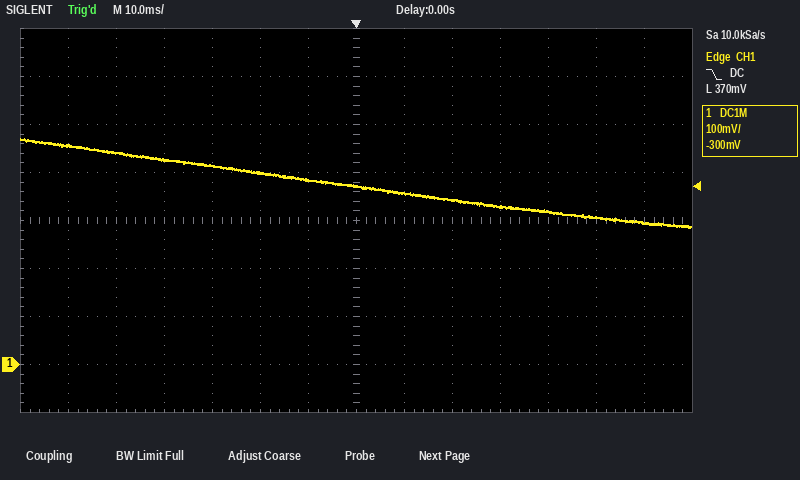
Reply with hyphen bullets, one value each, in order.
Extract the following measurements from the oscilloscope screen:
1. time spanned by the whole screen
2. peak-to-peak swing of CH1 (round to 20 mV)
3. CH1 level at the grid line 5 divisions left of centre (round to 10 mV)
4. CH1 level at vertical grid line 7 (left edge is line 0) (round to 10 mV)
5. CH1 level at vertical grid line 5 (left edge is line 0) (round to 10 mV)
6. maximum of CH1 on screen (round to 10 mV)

- 140 ms
- 180 mV
- 440 mV
- 370 mV
- 400 mV
- 470 mV
